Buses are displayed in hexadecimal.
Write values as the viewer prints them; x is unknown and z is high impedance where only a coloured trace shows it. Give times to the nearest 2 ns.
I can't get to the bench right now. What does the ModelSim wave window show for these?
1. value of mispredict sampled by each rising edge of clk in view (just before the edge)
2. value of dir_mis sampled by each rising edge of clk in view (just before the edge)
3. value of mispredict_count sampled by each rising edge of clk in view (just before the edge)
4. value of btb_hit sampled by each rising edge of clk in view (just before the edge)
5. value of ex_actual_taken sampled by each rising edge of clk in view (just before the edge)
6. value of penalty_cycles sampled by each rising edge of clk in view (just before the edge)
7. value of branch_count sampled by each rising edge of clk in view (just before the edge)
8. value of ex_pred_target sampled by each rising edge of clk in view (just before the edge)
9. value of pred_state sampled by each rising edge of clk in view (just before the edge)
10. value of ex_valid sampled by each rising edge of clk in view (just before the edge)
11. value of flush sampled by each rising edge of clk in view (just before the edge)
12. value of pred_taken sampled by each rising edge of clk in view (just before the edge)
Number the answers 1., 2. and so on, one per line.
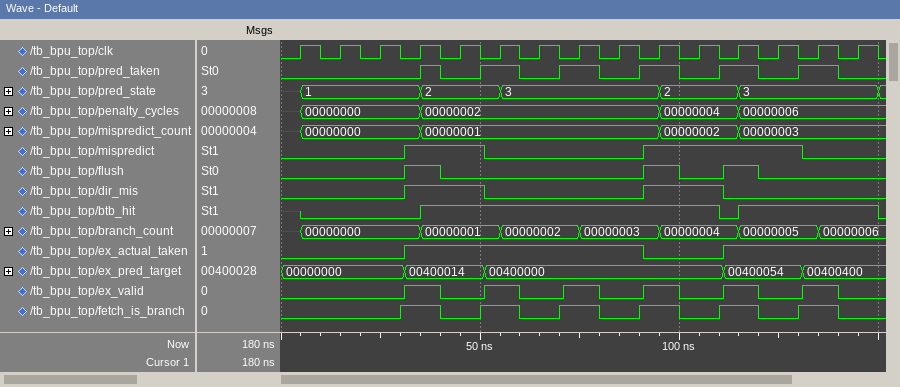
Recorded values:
1. 0 0 0 1 1 0 0 0 0 1 1 1 1 0 0
2. 0 0 0 1 1 0 0 0 0 1 1 0 0 0 0
3. x, 00000000, 00000000, 00000000, 00000001, 00000001, 00000001, 00000001, 00000001, 00000001, 00000002, 00000002, 00000003, 00000003, 00000003
4. x 0 0 0 1 1 1 1 1 1 1 0 1 1 1
5. 0 0 0 1 1 1 1 1 1 0 0 1 1 1 1
6. x, 00000000, 00000000, 00000000, 00000002, 00000002, 00000002, 00000002, 00000002, 00000002, 00000004, 00000004, 00000006, 00000006, 00000006
7. x, 00000000, 00000000, 00000000, 00000001, 00000001, 00000002, 00000002, 00000003, 00000003, 00000004, 00000004, 00000005, 00000005, 00000006
8. 00000000, 00000000, 00000000, 00400014, 00400014, 00400000, 00400000, 00400000, 00400000, 00400000, 00400000, 00400054, 00400054, 00400400, 00400400
9. x, 1, 1, 1, 2, 2, 3, 3, 3, 3, 2, 2, 3, 3, 3
10. 0 0 0 1 0 1 0 1 0 1 0 1 0 1 0
11. 0 0 0 1 0 0 0 0 0 1 0 1 0 0 0
12. 0 0 0 0 0 1 0 1 0 1 0 1 0 1 0
